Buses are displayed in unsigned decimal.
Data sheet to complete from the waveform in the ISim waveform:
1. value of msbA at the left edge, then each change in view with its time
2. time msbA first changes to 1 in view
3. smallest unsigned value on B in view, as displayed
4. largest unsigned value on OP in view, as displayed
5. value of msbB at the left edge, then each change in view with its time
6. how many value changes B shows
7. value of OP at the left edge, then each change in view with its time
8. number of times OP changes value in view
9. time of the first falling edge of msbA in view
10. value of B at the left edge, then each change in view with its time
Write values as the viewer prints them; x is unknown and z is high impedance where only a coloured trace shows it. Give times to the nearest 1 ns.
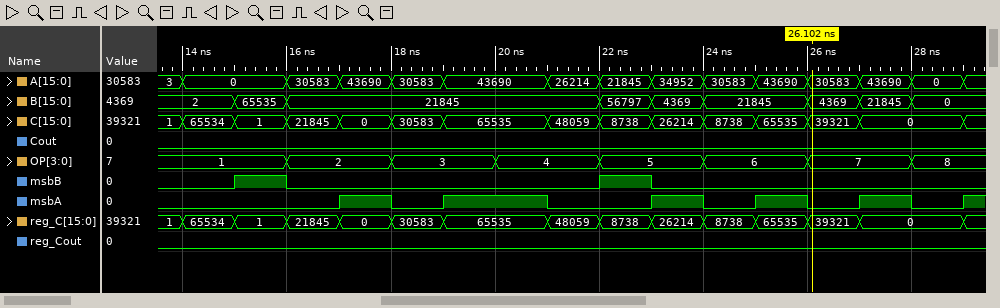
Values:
0, 1 at 17 ns, 0 at 18 ns, 1 at 19 ns, 0 at 21 ns, 1 at 23 ns, 0 at 24 ns, 1 at 25 ns, 0 at 26 ns, 1 at 27 ns, 0 at 28 ns, 1 at 29 ns
17 ns
0
8
0, 1 at 15 ns, 0 at 16 ns, 1 at 22 ns, 0 at 23 ns
8
1, 2 at 16 ns, 3 at 18 ns, 4 at 20 ns, 5 at 22 ns, 6 at 24 ns, 7 at 26 ns, 8 at 28 ns
7
18 ns
2, 65535 at 15 ns, 21845 at 16 ns, 56797 at 22 ns, 4369 at 23 ns, 21845 at 24 ns, 4369 at 26 ns, 21845 at 27 ns, 0 at 28 ns
